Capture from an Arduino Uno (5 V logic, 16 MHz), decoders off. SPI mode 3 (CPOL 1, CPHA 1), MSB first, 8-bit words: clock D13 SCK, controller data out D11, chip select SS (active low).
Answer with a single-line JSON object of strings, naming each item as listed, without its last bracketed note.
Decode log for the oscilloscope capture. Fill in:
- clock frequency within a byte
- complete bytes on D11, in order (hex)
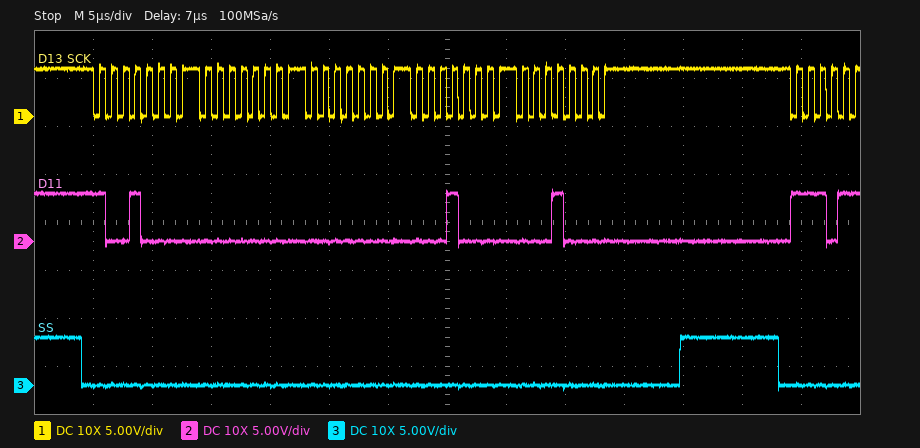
{"clock frequency within a byte": "1 MHz", "complete bytes on D11, in order": "90 00 00 10 10"}
